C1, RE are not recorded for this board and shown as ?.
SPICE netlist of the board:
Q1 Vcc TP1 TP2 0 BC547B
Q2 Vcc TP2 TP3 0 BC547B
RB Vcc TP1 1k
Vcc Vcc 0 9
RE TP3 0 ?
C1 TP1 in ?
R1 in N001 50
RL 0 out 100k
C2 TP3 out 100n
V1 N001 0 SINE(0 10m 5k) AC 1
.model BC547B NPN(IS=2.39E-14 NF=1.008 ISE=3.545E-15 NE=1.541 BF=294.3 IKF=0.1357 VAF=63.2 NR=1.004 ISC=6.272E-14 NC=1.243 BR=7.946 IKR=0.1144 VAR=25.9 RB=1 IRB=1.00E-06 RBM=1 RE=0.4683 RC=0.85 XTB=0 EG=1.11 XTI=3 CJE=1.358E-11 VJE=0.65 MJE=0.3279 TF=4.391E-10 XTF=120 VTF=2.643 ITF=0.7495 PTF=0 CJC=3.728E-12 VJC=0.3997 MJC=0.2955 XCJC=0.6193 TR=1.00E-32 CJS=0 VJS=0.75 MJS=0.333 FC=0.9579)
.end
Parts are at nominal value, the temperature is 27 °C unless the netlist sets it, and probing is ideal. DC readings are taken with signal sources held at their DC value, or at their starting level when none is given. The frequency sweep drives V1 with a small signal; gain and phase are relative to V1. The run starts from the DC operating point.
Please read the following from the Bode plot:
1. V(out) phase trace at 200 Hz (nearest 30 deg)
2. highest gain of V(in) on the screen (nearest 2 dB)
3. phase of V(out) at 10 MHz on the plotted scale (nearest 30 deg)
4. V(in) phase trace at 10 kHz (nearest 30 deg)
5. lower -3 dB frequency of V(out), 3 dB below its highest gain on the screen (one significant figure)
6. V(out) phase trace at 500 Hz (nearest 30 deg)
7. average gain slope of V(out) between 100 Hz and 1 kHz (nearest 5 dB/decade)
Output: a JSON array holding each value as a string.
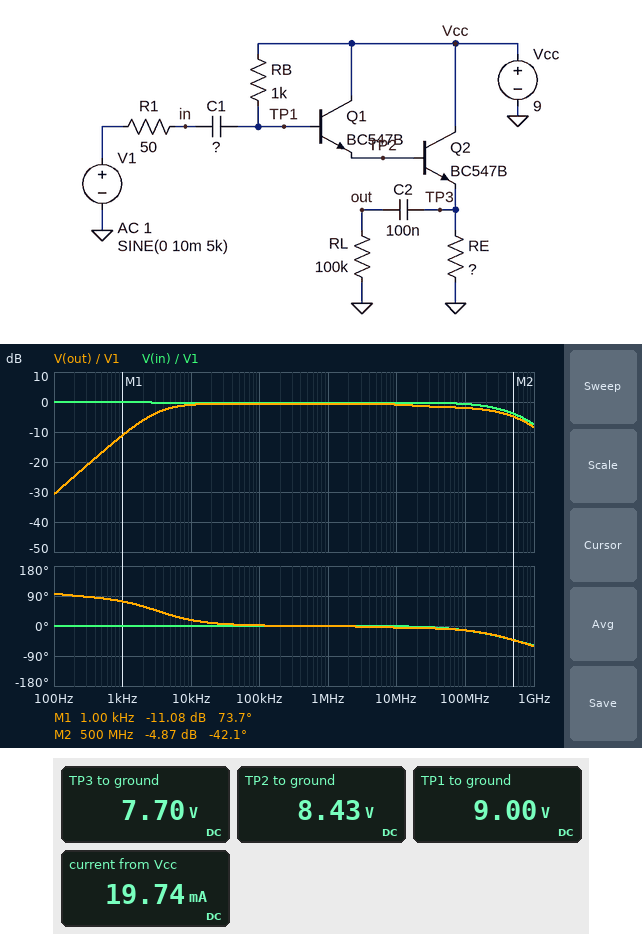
["90 deg", "0 dB", "0 deg", "0 deg", "3 kHz", "90 deg", "20 dB/decade"]
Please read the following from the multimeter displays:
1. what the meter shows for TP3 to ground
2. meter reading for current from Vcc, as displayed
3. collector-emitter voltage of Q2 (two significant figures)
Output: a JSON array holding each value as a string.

["7.70 V", "19.74 mA", "1.3 V"]
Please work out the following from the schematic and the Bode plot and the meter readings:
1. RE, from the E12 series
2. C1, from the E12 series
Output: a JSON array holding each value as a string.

["390 Ω", "47 nF"]
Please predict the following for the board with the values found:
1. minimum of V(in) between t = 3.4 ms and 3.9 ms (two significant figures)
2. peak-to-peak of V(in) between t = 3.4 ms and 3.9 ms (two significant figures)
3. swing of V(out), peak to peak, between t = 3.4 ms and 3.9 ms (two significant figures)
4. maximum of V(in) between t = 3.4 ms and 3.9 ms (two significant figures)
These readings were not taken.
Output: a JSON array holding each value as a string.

["-9.7 mV", "19 mV", "16 mV", "9.7 mV"]
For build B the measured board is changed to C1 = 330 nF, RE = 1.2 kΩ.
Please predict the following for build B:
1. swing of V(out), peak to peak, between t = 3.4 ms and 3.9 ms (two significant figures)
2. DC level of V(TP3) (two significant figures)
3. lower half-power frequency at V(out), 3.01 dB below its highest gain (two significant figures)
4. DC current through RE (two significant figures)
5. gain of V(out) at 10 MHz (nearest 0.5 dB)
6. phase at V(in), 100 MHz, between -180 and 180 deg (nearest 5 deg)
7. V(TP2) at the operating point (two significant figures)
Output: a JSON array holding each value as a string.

["19 mV", "7.8 V", "460 Hz", "6.5 mA", "-1.5 dB", "-10 deg", "8.5 V"]
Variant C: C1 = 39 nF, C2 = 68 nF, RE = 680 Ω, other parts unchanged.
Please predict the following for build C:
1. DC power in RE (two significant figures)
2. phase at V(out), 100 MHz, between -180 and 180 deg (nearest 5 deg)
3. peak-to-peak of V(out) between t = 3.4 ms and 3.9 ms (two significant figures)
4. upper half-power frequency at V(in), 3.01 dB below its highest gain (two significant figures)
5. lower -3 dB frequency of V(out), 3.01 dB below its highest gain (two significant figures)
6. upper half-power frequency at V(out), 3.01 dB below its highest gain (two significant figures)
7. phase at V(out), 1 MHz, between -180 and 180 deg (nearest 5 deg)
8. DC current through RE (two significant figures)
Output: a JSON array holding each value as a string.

["88 mW", "-10 deg", "15 mV", "430 MHz", "3.9 kHz", "360 MHz", "0 deg", "11 mA"]
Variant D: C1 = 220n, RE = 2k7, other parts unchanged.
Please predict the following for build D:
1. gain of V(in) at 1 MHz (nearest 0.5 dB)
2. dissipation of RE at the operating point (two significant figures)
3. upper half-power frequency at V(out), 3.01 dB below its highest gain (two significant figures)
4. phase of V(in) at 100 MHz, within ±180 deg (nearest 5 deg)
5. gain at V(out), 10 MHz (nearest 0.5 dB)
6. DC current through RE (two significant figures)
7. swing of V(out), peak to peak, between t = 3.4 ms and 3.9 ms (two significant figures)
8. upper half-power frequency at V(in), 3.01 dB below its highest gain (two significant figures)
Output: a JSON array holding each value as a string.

["-0.5 dB", "23 mW", "390 MHz", "-10 deg", "-1.5 dB", "2.9 mA", "19 mV", "460 MHz"]
